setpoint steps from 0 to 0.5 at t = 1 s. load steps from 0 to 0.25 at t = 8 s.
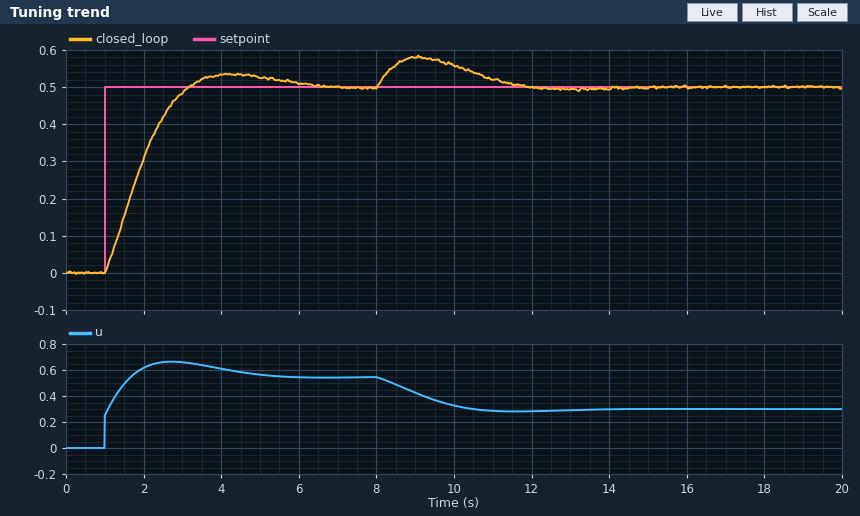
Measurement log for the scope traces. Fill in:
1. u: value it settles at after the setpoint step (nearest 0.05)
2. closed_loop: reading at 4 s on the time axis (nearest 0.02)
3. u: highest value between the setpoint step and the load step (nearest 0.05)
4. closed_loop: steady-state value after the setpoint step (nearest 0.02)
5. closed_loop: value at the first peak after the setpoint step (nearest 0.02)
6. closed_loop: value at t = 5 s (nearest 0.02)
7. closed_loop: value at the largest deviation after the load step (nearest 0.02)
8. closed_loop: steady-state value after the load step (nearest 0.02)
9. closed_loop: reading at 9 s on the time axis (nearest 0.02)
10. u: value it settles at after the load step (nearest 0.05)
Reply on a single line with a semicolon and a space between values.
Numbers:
0.55; 0.54; 0.65; 0.50; 0.54; 0.52; 0.58; 0.50; 0.58; 0.30
